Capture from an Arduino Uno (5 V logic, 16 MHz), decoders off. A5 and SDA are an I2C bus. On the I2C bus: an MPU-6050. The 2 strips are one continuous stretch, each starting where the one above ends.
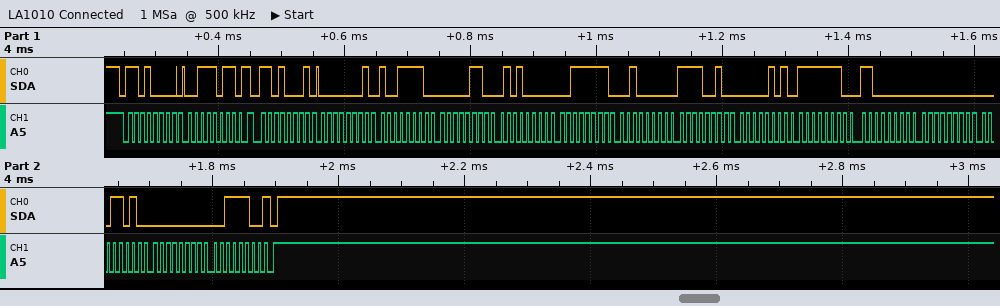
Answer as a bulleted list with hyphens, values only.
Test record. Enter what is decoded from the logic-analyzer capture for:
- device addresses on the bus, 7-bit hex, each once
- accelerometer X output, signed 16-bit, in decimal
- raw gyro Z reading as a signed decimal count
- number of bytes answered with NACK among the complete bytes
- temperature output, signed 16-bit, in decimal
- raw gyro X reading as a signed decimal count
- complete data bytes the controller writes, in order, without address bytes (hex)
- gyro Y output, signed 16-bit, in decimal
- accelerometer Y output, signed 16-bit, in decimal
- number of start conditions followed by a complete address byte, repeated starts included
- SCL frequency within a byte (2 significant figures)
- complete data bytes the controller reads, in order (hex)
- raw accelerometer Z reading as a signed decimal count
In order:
- 0x68
- 414
- 60
- 1
- -3579
- -320
- 3B
- 26
- 1616
- 2
- 100 kHz
- 01 9E 06 50 3F 20 F2 05 FE C0 00 1A 00 3C
- 16160
